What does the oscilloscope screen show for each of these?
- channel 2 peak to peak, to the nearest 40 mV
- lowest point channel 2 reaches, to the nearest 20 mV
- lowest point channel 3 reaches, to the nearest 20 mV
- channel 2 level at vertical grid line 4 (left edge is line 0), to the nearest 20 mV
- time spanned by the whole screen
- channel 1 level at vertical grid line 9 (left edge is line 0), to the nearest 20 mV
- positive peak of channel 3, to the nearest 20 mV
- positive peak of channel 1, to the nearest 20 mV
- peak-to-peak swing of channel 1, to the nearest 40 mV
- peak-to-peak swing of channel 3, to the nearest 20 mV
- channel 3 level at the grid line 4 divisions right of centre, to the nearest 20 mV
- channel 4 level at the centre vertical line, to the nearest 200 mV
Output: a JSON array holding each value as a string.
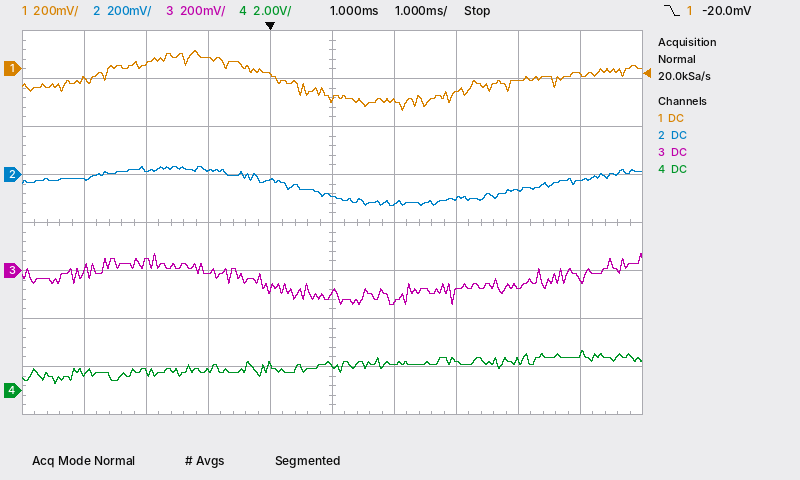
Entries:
["160 mV", "-120 mV", "-140 mV", "-20 mV", "10 ms", "-20 mV", "80 mV", "80 mV", "240 mV", "220 mV", "-40 mV", "1.0 V"]
